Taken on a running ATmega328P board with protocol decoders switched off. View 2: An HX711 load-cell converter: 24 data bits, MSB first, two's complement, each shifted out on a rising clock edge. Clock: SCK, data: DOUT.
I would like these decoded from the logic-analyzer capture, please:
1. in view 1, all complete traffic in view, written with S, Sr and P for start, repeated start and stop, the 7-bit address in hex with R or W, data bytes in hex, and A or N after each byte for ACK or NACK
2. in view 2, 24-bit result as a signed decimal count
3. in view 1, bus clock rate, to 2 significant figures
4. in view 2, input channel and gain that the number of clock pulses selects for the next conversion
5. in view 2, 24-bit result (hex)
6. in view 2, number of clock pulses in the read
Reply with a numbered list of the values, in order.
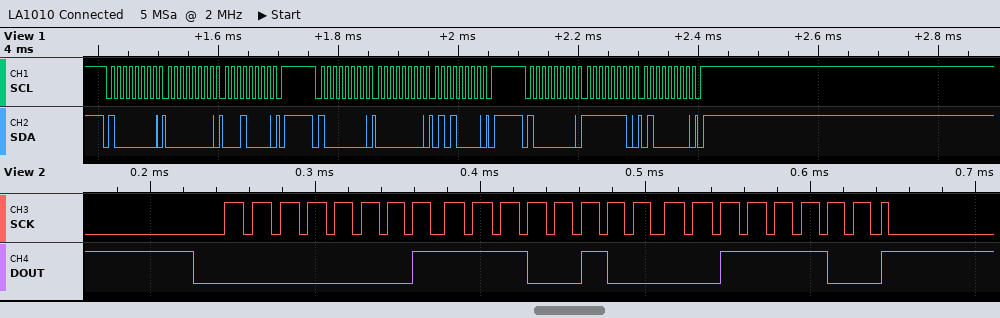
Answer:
1. S 40W A 00 A 10 A P S 40W A 00 A 50 A P S 40W A FE A 40 A P
2. 123964
3. 100 kHz
4. channel A, gain 128
5. 0x01E43C
6. 25
